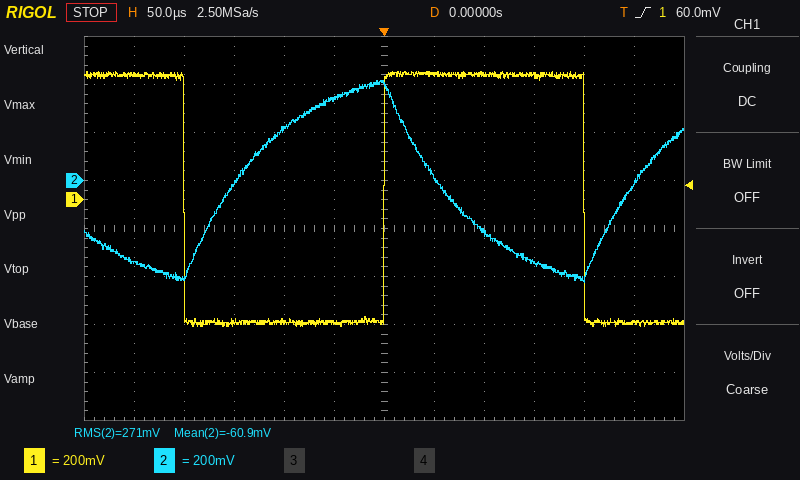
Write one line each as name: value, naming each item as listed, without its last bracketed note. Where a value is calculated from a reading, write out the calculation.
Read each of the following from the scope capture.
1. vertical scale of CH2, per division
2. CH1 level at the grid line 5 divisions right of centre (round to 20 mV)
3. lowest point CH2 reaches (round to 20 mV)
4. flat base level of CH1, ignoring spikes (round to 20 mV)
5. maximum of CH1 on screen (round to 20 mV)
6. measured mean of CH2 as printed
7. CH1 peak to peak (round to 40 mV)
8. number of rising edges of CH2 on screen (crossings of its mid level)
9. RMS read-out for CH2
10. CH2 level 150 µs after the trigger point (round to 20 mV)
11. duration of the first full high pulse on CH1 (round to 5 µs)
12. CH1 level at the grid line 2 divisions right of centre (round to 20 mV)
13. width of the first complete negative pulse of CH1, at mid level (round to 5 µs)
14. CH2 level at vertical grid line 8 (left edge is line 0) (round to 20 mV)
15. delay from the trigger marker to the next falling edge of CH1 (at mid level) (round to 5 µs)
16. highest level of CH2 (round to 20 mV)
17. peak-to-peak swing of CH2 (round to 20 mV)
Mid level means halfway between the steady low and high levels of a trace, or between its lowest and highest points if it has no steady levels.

vertical scale of CH2, per division: 200 mV
CH1 level at the grid line 5 divisions right of centre: -520 mV
lowest point CH2 reaches: -420 mV
flat base level of CH1, ignoring spikes: -520 mV
maximum of CH1 on screen: 540 mV
measured mean of CH2 as printed: -60.9 mV
CH1 peak to peak: 1.08 V
number of rising edges of CH2 on screen: 2
RMS read-out for CH2: 271 mV
CH2 level 150 µs after the trigger point: -340 mV
duration of the first full high pulse on CH1: 200 µs
CH1 level at the grid line 2 divisions right of centre: 520 mV
width of the first complete negative pulse of CH1, at mid level: 200 µs
CH2 level at vertical grid line 8 (left edge is line 0): -220 mV
delay from the trigger marker to the next falling edge of CH1 (at mid level): 200 µs
highest level of CH2: 420 mV
peak-to-peak swing of CH2: 420 mV − (-420 mV) = 840 mV
